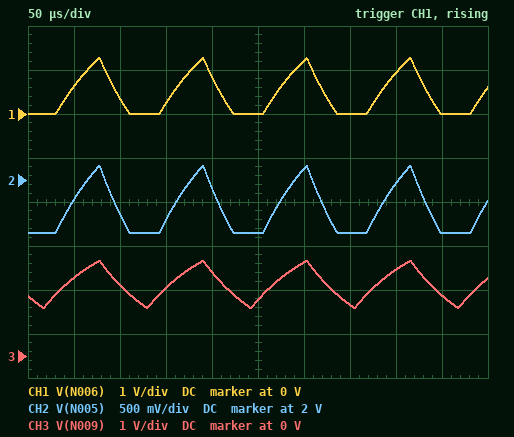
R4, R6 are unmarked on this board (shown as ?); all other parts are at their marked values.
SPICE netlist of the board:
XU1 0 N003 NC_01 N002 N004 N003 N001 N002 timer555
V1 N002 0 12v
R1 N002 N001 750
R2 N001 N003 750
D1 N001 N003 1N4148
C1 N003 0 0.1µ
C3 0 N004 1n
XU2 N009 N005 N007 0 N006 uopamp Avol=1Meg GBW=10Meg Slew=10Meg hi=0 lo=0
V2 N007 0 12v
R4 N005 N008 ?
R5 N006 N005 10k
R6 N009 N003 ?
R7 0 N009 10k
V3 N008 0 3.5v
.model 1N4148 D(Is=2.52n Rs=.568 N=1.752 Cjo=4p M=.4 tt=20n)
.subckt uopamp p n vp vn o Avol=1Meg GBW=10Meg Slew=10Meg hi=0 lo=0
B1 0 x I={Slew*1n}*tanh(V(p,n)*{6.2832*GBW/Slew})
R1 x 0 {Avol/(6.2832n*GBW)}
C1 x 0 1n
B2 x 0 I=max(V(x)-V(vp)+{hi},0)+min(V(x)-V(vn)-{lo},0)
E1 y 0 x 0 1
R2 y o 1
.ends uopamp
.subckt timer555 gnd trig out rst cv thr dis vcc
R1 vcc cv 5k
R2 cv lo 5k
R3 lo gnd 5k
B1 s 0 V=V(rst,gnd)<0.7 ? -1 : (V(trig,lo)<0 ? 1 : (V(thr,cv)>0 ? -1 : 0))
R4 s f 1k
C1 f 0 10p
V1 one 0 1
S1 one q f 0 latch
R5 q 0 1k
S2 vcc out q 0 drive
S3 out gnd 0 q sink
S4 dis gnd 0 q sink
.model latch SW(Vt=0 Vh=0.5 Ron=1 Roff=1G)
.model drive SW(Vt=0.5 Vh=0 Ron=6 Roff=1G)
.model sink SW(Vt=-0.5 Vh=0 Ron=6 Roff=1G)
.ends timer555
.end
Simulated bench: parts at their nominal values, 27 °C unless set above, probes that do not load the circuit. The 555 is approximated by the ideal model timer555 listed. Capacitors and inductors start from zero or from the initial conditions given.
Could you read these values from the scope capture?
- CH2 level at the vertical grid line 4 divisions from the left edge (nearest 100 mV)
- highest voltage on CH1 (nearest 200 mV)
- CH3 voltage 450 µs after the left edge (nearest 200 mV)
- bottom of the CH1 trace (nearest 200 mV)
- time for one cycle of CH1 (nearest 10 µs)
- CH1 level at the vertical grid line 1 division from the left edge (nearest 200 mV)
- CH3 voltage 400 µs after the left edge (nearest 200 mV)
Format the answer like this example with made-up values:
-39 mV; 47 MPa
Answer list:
1.9 V; 1.2 V; 1.4 V; 0 V; 110 µs; 600 mV; 2.0 V
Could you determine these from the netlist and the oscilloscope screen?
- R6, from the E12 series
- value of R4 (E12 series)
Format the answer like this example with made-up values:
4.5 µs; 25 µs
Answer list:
27 kΩ; 15 kΩ
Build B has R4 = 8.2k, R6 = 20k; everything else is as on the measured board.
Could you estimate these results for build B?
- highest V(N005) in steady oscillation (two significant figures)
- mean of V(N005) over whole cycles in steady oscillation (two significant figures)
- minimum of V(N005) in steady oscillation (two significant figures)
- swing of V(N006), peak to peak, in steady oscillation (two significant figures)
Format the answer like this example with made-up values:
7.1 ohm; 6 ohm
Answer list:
2.7 V; 2.1 V; 1.9 V; 1.7 V
